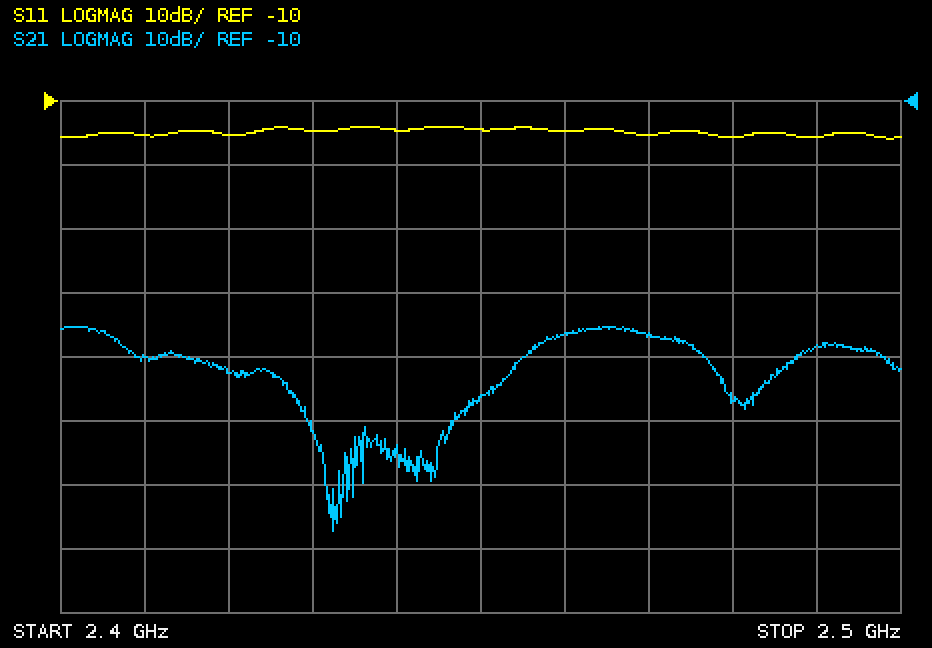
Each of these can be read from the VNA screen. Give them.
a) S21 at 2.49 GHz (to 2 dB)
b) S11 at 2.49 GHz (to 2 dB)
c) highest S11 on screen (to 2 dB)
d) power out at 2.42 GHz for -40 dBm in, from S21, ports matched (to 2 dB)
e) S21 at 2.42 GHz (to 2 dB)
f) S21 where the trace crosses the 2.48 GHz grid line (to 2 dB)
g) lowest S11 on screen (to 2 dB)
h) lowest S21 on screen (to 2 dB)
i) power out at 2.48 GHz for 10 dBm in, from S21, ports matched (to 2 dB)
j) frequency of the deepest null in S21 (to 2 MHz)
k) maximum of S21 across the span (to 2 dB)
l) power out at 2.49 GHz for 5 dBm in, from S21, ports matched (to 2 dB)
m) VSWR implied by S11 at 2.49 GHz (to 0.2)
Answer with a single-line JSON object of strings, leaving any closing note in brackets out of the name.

{"S21 at 2.49 GHz": "-48 dB", "S11 at 2.49 GHz": "-16 dB", "highest S11 on screen": "-14 dB", "power out at 2.42 GHz for -40 dBm in, from S21, ports matched": "-92 dBm", "S21 at 2.42 GHz": "-52 dB", "S21 where the trace crosses the 2.48 GHz grid line": "-56 dB", "lowest S11 on screen": "-16 dB", "lowest S21 on screen": "-78 dB", "power out at 2.48 GHz for 10 dBm in, from S21, ports matched": "-46 dBm", "frequency of the deepest null in S21": "2.432 GHz", "maximum of S21 across the span": "-46 dB", "power out at 2.49 GHz for 5 dBm in, from S21, ports matched": "-44 dBm", "VSWR implied by S11 at 2.49 GHz": "1.4"}
